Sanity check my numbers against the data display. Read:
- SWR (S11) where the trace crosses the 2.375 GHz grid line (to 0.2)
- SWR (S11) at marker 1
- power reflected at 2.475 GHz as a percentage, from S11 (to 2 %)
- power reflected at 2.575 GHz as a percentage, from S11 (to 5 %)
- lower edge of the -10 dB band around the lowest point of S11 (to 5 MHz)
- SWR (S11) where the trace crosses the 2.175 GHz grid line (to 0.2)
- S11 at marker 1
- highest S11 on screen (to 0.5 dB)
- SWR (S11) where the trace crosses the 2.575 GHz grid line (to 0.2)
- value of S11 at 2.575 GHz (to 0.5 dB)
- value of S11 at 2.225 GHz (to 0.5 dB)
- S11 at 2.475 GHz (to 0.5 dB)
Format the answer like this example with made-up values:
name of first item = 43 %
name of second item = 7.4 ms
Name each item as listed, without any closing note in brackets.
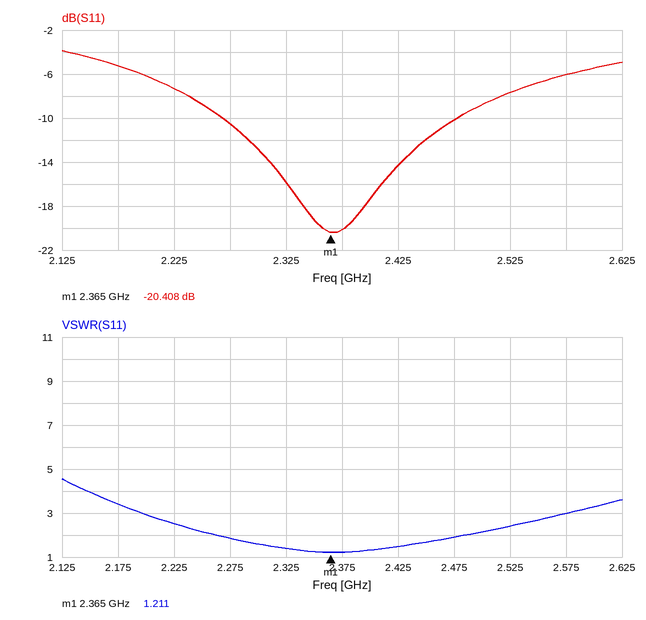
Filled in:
SWR (S11) where the trace crosses the 2.375 GHz grid line = 1.2
SWR (S11) at marker 1 = 1.211
power reflected at 2.475 GHz as a percentage, from S11 = 10 %
power reflected at 2.575 GHz as a percentage, from S11 = 25 %
lower edge of the -10 dB band around the lowest point of S11 = 2.270 GHz
SWR (S11) where the trace crosses the 2.175 GHz grid line = 3.4
S11 at marker 1 = -20.408 dB
highest S11 on screen = -4.0 dB
SWR (S11) where the trace crosses the 2.575 GHz grid line = 3.0
value of S11 at 2.575 GHz = -6.0 dB
value of S11 at 2.225 GHz = -7.5 dB
S11 at 2.475 GHz = -10.0 dB
